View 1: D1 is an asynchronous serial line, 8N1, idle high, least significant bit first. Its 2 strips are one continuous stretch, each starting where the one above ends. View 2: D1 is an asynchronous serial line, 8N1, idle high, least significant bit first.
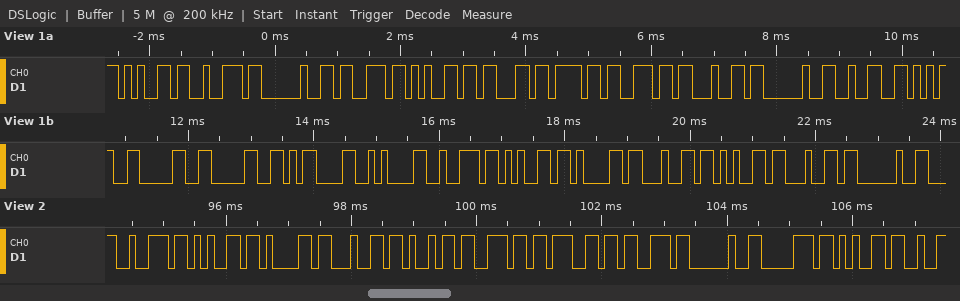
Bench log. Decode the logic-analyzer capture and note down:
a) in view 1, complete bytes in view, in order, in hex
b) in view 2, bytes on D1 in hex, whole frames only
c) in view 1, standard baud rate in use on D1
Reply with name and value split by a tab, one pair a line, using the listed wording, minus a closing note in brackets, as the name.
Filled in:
in view 1, complete bytes in view, in order, in hex	65 72 20 73 65 63 6F 6E 64 20 32 35 30 30 0D 0A 72 65 61 64 65 64 20
in view 2, bytes on D1 in hex, whole frames only	0x72 0x65 0x61 0x64 0x69 0x6E 0x67 0x73 0x20 0x70 0x65
in view 1, standard baud rate in use on D1	9600 baud
